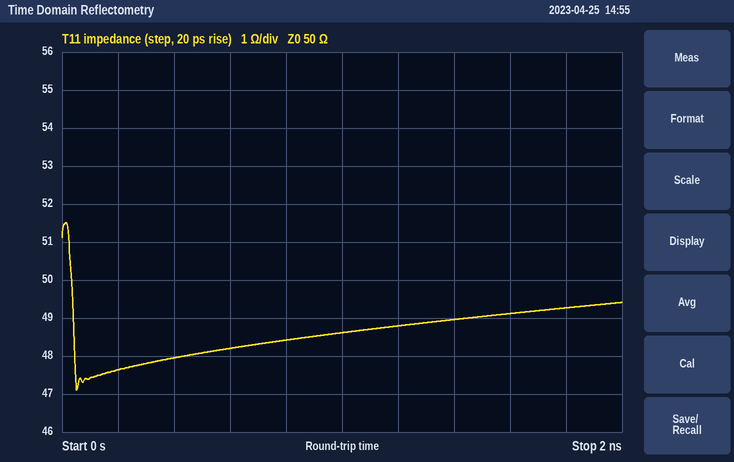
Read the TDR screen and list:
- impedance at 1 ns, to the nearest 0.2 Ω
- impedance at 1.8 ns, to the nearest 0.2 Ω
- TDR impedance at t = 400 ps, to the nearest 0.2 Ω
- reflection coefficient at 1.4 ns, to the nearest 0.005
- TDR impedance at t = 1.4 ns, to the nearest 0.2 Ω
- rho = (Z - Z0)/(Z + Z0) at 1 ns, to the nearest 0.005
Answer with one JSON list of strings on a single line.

["48.6 Ω", "49.2 Ω", "48.0 Ω", "-0.010", "49.0 Ω", "-0.015"]
